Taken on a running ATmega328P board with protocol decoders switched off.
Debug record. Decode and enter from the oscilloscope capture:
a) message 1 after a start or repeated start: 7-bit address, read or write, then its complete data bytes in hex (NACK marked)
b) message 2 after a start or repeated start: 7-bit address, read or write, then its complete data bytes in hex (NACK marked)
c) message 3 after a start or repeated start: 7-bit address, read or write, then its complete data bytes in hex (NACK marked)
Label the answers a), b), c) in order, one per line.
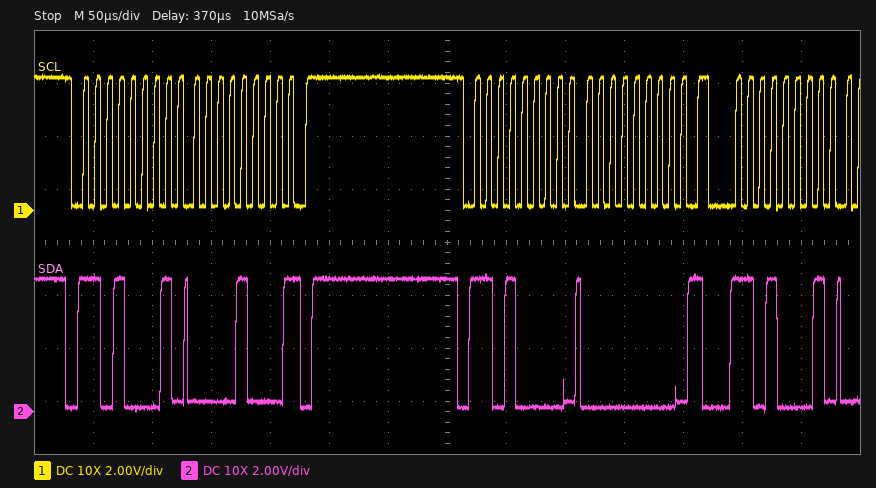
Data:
a) 0x68 read: 08 NACK
b) 0x68 write: 00
c) 0x68 read
